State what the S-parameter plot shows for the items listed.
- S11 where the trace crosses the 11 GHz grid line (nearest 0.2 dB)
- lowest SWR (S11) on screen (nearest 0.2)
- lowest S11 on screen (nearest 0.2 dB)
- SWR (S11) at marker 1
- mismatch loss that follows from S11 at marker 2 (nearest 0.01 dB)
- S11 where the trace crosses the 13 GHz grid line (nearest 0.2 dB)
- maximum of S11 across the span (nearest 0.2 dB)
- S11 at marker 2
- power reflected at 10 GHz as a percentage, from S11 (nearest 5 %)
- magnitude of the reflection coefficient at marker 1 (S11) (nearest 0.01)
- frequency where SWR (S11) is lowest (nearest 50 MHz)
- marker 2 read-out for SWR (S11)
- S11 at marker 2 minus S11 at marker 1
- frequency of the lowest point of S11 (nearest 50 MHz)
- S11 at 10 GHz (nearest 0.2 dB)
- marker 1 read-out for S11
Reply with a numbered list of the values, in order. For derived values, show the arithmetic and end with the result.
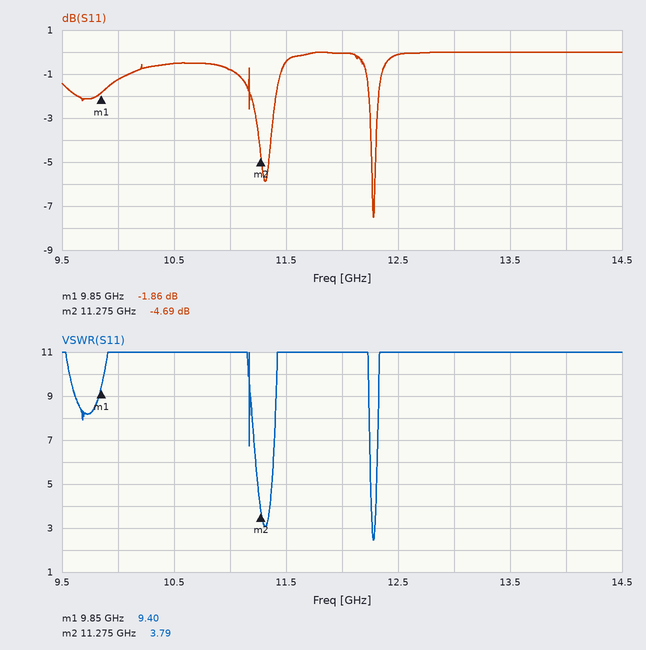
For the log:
1. -0.8 dB
2. 2.4
3. -7.6 dB
4. 9.40
5. −10 log10(1 − 10^(-4.69/10)) ≈ 1.80 dB
6. 0.0 dB
7. 0.0 dB
8. -4.69 dB
9. 10^(-1.2/10) ≈ 75.9 %, so 75 % to the nearest 5 %
10. 10^(-1.86/20) ≈ 0.81
11. 12.30 GHz
12. 3.79
13. -4.69 − (-1.86) = -2.83 dB
14. 12.30 GHz
15. -1.2 dB
16. -1.86 dB
